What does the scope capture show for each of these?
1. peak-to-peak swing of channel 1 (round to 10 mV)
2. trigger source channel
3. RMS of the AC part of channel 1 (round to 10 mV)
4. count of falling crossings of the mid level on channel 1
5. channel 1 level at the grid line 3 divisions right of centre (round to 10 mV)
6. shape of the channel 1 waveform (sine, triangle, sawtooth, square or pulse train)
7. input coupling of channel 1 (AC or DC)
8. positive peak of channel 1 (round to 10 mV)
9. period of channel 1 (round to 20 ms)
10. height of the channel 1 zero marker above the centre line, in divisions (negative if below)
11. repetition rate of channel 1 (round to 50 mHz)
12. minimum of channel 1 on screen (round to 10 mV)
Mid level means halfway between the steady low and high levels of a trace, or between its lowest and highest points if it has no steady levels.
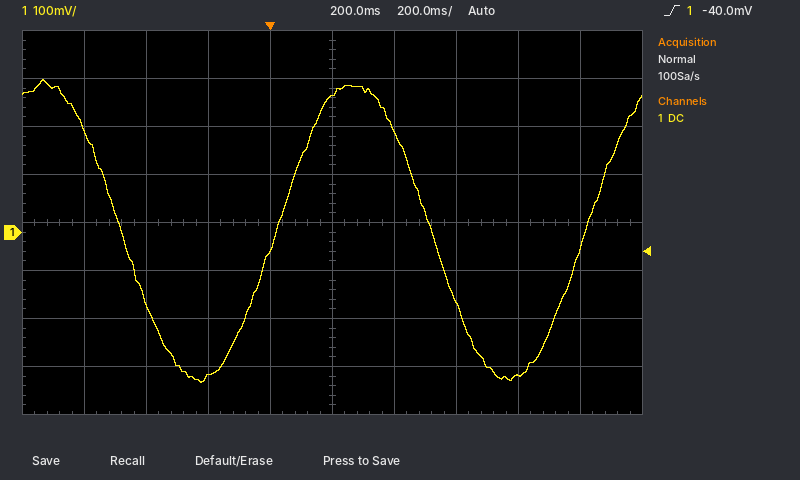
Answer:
630 mV
channel 1
220 mV
2
-300 mV
sine
DC
320 mV
1.00 s
-0.2 div
1.00 Hz
-310 mV
